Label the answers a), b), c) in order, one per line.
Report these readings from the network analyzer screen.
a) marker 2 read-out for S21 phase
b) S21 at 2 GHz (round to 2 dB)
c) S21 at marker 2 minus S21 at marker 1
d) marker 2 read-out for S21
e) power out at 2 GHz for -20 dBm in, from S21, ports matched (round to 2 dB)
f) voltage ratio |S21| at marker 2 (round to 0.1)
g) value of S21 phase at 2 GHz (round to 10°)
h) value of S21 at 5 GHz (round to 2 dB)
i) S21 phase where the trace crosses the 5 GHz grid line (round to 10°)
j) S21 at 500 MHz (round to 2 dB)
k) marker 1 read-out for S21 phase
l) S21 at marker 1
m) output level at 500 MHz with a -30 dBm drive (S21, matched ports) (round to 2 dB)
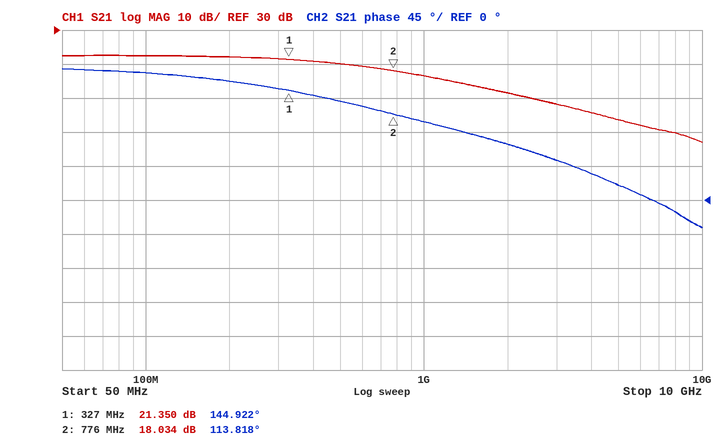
a) 113.818°
b) 12 dB
c) -3.316 dB
d) 18.034 dB
e) -8 dBm
f) 8.0
g) 70°
h) 4 dB
i) 20°
j) 20 dB
k) 144.922°
l) 21.350 dB
m) -10 dBm
